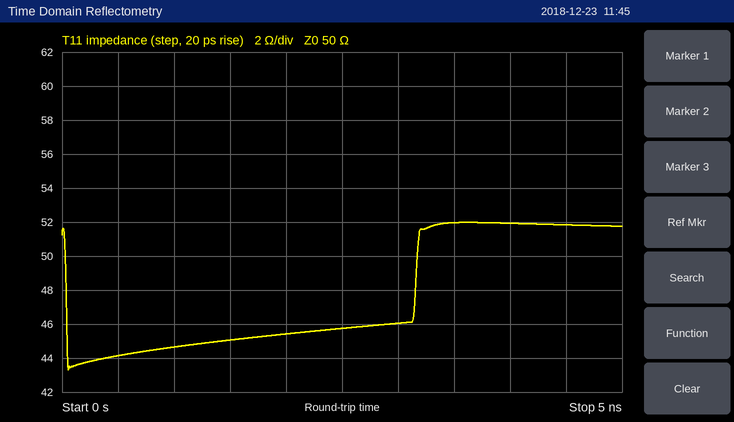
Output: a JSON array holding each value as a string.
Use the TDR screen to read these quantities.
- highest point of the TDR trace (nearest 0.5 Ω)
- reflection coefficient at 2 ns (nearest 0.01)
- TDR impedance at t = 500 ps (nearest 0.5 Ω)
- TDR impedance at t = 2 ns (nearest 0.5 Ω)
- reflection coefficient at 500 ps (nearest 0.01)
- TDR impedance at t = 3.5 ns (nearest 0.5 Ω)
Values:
["52.0 Ω", "-0.05", "44.0 Ω", "45.5 Ω", "-0.06", "52.0 Ω"]
